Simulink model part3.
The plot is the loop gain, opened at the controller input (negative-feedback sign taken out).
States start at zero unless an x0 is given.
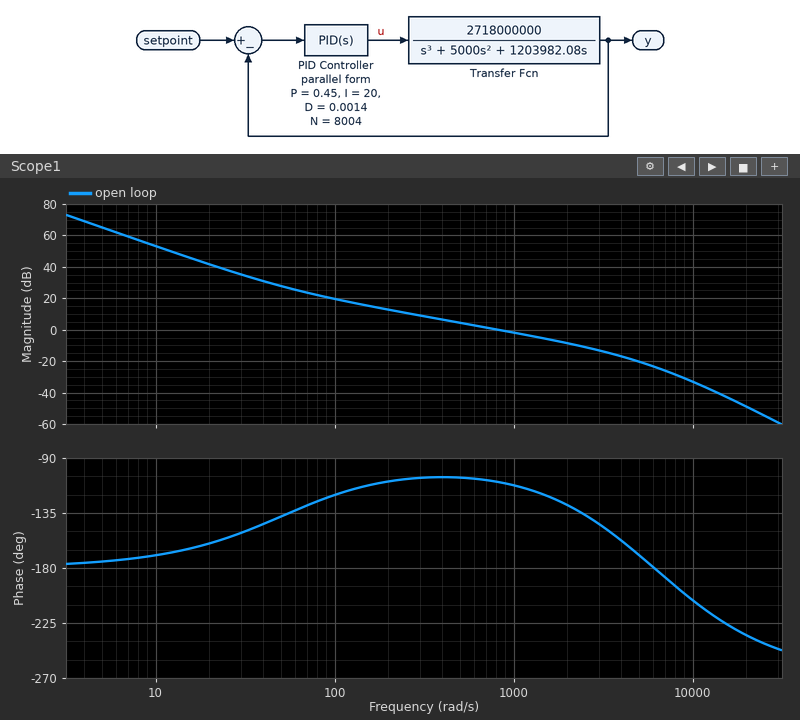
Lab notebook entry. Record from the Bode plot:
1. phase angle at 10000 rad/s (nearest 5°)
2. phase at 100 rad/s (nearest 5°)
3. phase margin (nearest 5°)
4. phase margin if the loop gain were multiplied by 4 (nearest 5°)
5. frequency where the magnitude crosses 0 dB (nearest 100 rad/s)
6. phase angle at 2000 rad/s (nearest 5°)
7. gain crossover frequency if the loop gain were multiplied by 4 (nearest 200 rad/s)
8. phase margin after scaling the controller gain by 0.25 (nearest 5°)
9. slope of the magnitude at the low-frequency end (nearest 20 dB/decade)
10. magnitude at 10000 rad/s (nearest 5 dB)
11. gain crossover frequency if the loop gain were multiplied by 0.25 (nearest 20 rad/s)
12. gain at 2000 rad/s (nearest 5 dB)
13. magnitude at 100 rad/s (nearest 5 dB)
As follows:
-205°
-120°
70°
40°
800 rad/s
-130°
2800 rad/s
70°
-40 dB/decade
-35 dB
220 rad/s
-10 dB
20 dB
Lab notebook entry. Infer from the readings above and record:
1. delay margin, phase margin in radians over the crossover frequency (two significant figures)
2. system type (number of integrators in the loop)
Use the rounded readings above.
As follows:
0.0015 s
2
